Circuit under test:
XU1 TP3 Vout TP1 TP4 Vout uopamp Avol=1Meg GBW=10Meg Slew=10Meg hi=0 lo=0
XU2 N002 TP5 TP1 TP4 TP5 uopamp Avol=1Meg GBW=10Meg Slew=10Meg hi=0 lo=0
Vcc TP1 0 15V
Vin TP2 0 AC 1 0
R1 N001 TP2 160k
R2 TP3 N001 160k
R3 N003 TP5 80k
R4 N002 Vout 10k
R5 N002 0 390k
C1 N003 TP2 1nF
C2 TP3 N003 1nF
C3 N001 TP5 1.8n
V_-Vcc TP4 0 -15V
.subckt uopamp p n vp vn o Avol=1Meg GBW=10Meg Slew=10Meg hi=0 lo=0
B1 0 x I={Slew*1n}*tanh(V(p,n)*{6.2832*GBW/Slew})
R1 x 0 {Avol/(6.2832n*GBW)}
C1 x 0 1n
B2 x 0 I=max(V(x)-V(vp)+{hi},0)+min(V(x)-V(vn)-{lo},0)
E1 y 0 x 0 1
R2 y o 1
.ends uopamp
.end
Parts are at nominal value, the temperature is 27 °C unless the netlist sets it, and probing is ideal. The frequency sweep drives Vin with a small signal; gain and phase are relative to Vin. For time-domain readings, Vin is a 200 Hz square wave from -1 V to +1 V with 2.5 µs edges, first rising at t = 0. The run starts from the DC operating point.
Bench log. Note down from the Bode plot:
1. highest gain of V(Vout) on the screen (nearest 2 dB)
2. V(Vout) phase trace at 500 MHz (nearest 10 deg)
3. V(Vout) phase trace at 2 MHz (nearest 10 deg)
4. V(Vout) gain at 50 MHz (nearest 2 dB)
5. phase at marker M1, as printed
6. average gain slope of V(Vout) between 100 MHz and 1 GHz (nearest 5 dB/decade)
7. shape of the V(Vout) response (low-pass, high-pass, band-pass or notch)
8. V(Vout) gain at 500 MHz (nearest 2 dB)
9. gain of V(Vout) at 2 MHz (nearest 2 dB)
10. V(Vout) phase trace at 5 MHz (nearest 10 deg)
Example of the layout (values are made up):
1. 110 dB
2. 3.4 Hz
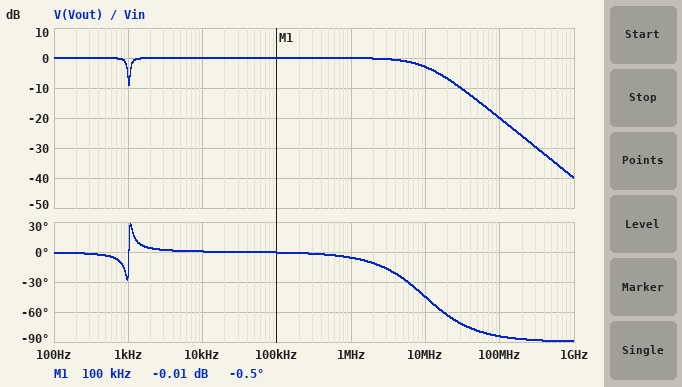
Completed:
1. 0 dB
2. -90 deg
3. -10 deg
4. -14 dB
5. -0.5 deg
6. -20 dB/decade
7. low-pass
8. -34 dB
9. 0 dB
10. -30 deg
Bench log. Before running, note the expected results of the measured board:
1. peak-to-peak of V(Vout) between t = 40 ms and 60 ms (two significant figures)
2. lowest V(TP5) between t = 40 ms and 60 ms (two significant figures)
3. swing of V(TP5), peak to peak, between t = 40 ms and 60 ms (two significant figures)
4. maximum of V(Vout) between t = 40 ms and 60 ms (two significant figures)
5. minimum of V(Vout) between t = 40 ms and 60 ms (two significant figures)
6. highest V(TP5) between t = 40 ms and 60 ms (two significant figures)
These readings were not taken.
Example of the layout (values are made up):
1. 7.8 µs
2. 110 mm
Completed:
1. 2.4 V
2. -1.2 V
3. 2.3 V
4. 1.2 V
5. -1.2 V
6. 1.2 V
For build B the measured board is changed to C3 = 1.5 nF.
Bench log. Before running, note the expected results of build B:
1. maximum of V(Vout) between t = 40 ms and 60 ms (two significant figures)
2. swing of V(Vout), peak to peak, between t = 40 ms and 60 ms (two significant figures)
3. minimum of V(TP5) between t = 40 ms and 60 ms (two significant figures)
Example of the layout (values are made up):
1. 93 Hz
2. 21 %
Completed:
1. 1.1 V
2. 2.2 V
3. -1.1 V
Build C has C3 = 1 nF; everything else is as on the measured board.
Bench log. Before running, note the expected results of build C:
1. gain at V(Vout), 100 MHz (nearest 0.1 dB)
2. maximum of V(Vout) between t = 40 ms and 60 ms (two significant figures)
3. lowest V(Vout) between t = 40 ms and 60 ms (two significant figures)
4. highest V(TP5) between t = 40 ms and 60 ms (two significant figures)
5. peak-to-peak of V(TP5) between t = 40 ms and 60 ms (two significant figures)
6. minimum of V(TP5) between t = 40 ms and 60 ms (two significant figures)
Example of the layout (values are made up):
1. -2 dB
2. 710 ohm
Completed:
1. -20.0 dB
2. 1.1 V
3. -1.1 V
4. 1.0 V
5. 2.1 V
6. -1.0 V
